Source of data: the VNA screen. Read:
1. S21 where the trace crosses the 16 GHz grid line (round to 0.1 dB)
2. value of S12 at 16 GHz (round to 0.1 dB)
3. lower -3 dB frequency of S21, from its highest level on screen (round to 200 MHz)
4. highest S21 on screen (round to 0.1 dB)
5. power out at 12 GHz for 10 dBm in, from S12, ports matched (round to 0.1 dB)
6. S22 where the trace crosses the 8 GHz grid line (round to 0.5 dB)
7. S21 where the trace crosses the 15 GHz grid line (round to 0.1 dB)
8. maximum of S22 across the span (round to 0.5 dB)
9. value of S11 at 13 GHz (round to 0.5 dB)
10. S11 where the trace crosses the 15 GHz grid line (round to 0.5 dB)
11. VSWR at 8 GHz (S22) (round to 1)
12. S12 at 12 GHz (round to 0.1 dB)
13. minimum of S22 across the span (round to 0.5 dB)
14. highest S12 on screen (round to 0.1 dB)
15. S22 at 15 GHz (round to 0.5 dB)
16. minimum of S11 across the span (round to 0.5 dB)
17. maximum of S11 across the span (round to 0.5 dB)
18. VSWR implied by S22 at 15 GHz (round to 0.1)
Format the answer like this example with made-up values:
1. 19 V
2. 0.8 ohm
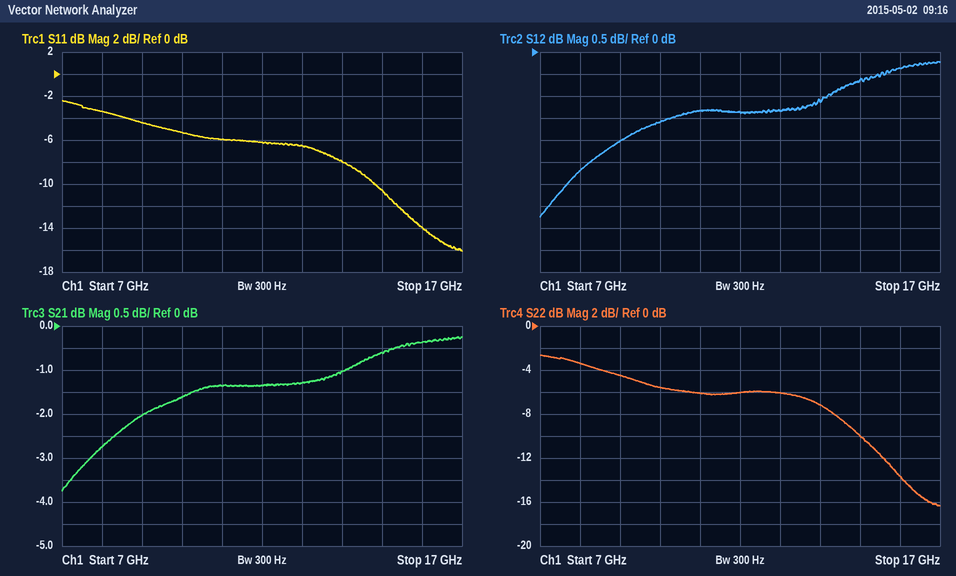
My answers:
1. -0.4 dB
2. -0.4 dB
3. 7.4 GHz
4. -0.2 dB
5. 8.6 dBm
6. -3.5 dB
7. -0.6 dB
8. -2.5 dB
9. -6.5 dB
10. -10.5 dB
11. 5
12. -1.4 dB
13. -16.5 dB
14. -0.2 dB
15. -10.0 dB
16. -16.0 dB
17. -2.5 dB
18. 1.9
